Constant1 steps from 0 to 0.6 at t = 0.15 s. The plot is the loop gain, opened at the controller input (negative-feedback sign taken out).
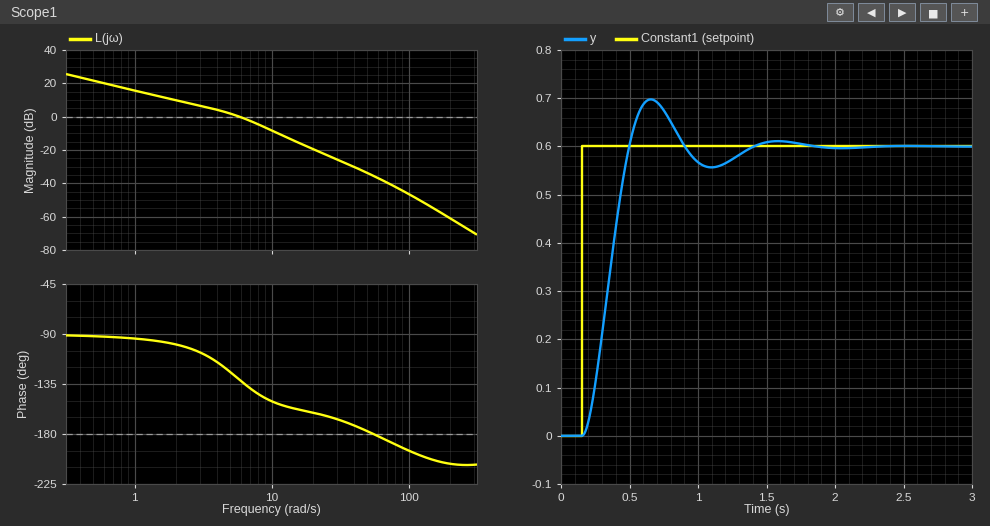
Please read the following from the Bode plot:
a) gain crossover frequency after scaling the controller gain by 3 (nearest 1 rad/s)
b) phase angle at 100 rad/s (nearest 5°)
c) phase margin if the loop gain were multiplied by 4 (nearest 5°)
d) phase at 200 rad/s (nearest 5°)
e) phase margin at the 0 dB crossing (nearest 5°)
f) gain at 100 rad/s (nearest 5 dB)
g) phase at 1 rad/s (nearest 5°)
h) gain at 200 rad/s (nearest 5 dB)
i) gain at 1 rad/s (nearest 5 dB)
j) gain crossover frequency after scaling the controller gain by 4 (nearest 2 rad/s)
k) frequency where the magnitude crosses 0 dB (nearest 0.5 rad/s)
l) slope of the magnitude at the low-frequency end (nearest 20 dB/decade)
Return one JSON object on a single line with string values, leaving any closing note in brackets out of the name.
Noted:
{"gain crossover frequency after scaling the controller gain by 3": "11 rad/s", "phase angle at 100 rad/s": "-195°", "phase margin if the loop gain were multiplied by 4": "25°", "phase at 200 rad/s": "-205°", "phase margin at the 0 dB crossing": "50°", "gain at 100 rad/s": "-45 dB", "phase at 1 rad/s": "-95°", "gain at 200 rad/s": "-60 dB", "gain at 1 rad/s": "15 dB", "gain crossover frequency after scaling the controller gain by 4": "12 rad/s", "frequency where the magnitude crosses 0 dB": "6.0 rad/s", "slope of the magnitude at the low-frequency end": "-20 dB/decade"}
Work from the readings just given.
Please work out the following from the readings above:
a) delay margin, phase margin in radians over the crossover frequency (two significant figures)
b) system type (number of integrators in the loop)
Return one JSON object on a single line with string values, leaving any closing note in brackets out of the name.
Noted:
{"delay margin, phase margin in radians over the crossover frequency": "0.15 s", "system type": "1"}
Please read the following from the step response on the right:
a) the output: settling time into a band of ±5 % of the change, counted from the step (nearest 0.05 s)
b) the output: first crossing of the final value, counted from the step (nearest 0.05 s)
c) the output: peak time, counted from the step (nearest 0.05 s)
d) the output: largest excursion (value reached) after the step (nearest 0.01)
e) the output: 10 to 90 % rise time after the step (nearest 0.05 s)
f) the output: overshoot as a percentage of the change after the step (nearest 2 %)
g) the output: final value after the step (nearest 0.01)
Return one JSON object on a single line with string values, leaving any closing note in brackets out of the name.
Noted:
{"the output: settling time into a band of ±5 % of the change, counted from the step": "1.10 s", "the output: first crossing of the final value, counted from the step": "0.35 s", "the output: peak time, counted from the step": "0.50 s", "the output: largest excursion (value reached) after the step": "0.70", "the output: 10 to 90 % rise time after the step": "0.25 s", "the output: overshoot as a percentage of the change after the step": "16 %", "the output: final value after the step": "0.60"}
